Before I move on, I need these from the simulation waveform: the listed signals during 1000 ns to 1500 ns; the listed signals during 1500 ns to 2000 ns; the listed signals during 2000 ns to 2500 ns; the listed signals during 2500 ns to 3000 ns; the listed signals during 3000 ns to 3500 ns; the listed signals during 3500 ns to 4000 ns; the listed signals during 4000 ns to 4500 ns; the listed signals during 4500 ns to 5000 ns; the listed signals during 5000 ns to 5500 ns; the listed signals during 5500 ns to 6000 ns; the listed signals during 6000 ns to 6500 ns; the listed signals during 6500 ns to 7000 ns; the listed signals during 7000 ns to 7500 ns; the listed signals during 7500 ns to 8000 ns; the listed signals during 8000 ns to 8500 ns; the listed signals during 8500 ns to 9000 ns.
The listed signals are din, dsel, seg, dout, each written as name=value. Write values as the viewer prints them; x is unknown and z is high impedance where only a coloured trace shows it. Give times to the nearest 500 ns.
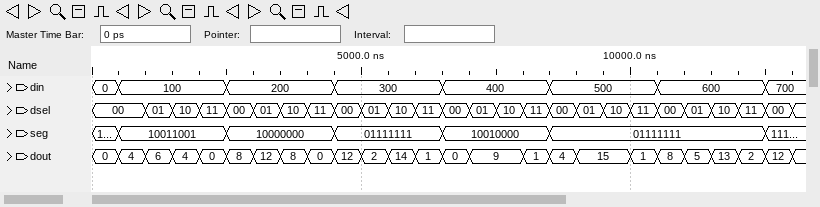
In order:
din=100, dsel=01, seg=10011001, dout=6
din=100, dsel=10, seg=10011001, dout=4
din=100, dsel=11, seg=10011001, dout=0
din=200, dsel=00, seg=10000000, dout=8
din=200, dsel=01, seg=10000000, dout=12
din=200, dsel=10, seg=10000000, dout=8
din=200, dsel=11, seg=10000000, dout=0
din=300, dsel=00, seg=01111111, dout=12
din=300, dsel=01, seg=01111111, dout=2
din=300, dsel=10, seg=01111111, dout=14
din=300, dsel=11, seg=01111111, dout=1
din=400, dsel=00, seg=10010000, dout=0
din=400, dsel=01, seg=10010000, dout=9
din=400, dsel=10, seg=10010000, dout=9
din=400, dsel=11, seg=10010000, dout=1
din=500, dsel=00, seg=01111111, dout=4
